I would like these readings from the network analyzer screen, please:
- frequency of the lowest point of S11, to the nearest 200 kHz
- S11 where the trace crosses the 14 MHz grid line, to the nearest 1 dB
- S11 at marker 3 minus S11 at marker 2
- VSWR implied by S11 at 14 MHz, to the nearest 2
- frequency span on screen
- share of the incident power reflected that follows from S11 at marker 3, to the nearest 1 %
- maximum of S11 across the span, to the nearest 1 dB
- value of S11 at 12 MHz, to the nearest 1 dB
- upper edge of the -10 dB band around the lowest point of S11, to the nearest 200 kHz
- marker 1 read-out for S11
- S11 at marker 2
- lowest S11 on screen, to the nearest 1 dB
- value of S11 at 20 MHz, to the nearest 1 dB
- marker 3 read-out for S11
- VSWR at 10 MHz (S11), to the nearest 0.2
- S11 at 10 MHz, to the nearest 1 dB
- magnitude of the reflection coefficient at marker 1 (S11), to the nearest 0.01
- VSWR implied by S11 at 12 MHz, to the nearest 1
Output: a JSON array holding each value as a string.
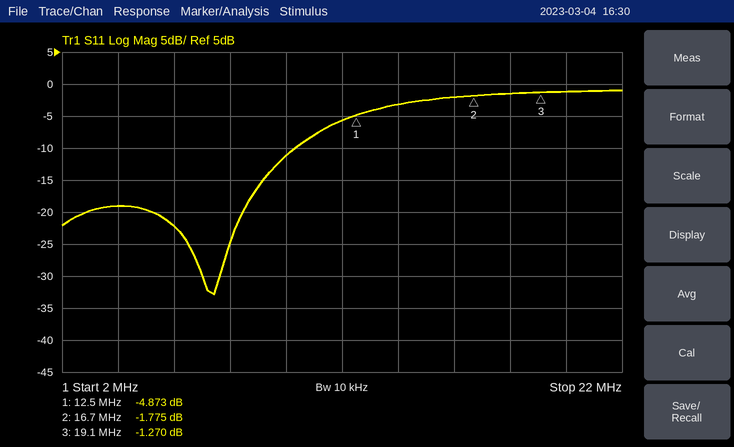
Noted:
["7.4 MHz", "-3 dB", "0.505 dB", "6", "20 MHz", "75 %", "-1 dB", "-6 dB", "10.4 MHz", "-4.873 dB", "-1.775 dB", "-33 dB", "-1 dB", "-1.270 dB", "1.8", "-11 dB", "0.57", "3"]
